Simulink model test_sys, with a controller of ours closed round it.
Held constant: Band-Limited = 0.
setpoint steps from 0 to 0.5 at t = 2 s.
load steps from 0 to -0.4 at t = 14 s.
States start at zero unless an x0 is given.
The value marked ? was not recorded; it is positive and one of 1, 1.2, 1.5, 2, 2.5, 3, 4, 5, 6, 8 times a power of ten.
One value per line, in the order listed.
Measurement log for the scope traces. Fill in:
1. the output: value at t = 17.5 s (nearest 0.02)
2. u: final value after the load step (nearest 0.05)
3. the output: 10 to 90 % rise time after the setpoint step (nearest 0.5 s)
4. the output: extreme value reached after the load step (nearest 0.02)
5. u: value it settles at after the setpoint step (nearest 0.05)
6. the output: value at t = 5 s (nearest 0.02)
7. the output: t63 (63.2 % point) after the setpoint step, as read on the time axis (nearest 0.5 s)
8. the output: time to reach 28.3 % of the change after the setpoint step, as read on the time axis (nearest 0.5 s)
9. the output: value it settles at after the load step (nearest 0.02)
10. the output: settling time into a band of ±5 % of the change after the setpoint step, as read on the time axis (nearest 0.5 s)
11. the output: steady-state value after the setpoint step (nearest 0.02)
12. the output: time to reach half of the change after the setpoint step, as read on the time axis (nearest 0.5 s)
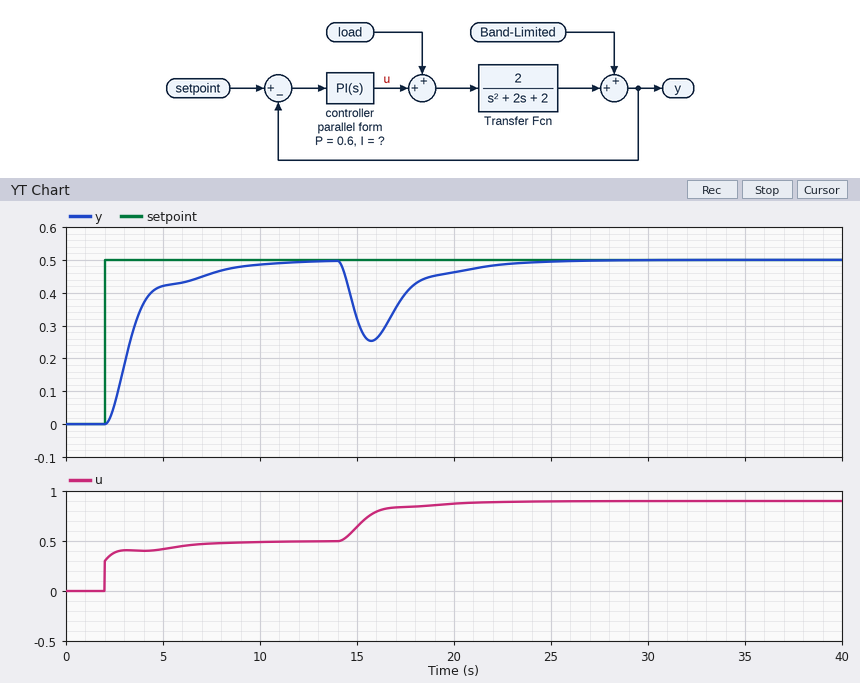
0.40
0.90
4.5 s
0.26
0.50
0.42
3.5 s
3.0 s
0.50
8.5 s
0.50
3.5 s
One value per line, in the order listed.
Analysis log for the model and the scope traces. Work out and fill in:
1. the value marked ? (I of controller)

0.5
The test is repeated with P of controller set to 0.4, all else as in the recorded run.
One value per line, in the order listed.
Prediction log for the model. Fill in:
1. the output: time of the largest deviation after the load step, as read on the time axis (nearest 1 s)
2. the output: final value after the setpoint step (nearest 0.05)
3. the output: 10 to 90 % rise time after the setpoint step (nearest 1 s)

16 s
0.50
3 s
